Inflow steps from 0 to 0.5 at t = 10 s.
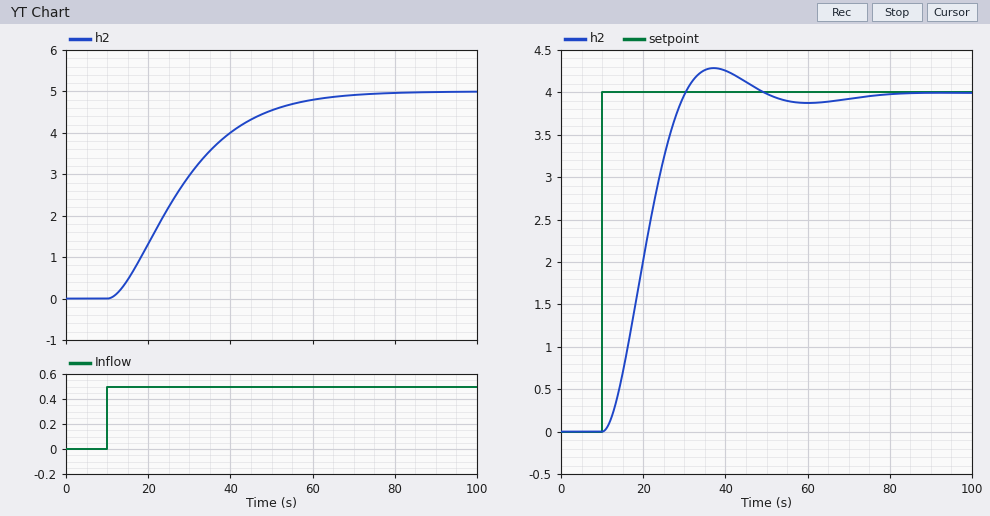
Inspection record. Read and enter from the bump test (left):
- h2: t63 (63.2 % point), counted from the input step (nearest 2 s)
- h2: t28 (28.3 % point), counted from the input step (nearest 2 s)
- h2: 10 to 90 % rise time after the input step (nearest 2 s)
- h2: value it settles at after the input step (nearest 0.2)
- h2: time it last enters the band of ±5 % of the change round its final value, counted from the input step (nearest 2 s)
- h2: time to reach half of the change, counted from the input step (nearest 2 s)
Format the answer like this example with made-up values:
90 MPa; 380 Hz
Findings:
22 s; 10 s; 34 s; 5.0; 48 s; 16 s
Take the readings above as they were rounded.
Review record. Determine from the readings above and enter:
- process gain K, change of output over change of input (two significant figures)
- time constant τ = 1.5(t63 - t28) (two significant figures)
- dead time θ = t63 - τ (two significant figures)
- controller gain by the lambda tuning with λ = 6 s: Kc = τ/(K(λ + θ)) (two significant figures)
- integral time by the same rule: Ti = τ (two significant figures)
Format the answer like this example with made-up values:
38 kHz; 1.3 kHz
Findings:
10; 18 s; 4.0 s; 0.18; 18 s
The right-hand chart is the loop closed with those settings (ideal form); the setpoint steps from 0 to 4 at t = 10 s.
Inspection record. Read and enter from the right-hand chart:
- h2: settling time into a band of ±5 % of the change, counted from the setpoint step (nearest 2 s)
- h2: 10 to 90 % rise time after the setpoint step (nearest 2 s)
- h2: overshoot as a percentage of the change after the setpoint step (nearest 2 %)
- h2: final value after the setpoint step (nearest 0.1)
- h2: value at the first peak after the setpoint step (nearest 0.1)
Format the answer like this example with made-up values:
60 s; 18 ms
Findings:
32 s; 14 s; 8 %; 4.0; 4.3
